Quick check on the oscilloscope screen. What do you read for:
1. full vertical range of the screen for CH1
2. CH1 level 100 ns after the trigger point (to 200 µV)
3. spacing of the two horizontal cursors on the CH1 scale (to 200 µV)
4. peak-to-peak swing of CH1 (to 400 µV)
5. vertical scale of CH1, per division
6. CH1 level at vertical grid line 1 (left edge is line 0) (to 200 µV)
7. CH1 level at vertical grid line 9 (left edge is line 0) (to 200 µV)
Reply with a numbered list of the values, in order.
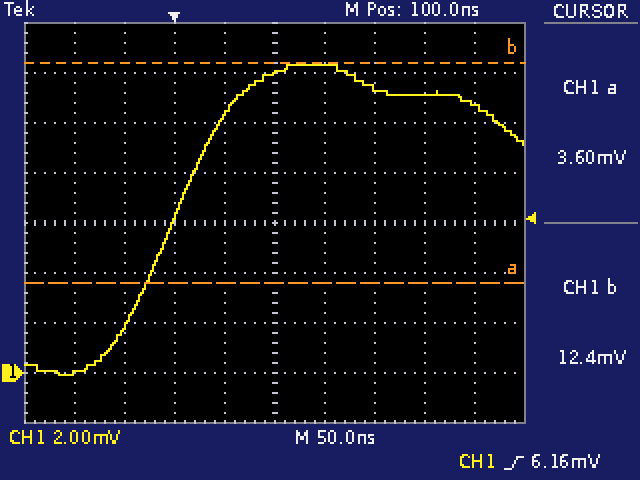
1. 16 mV
2. 12.0 mV
3. 8.8 mV
4. 12.4 mV
5. 2 mV
6. 0.0 mV
7. 10.8 mV
